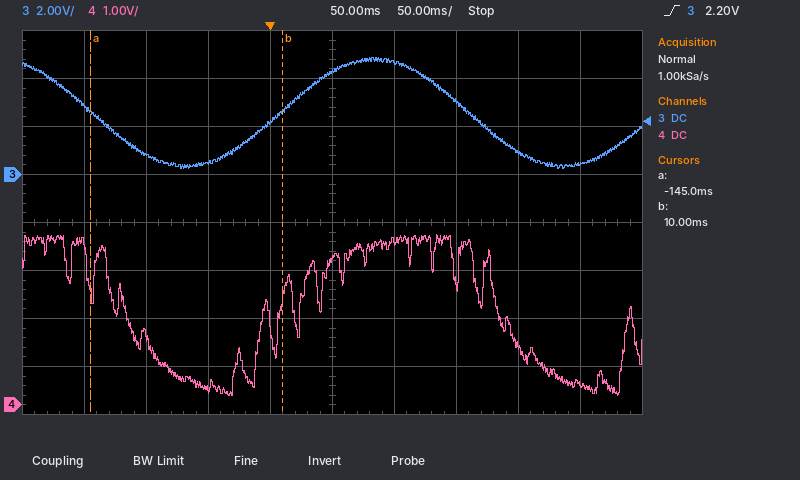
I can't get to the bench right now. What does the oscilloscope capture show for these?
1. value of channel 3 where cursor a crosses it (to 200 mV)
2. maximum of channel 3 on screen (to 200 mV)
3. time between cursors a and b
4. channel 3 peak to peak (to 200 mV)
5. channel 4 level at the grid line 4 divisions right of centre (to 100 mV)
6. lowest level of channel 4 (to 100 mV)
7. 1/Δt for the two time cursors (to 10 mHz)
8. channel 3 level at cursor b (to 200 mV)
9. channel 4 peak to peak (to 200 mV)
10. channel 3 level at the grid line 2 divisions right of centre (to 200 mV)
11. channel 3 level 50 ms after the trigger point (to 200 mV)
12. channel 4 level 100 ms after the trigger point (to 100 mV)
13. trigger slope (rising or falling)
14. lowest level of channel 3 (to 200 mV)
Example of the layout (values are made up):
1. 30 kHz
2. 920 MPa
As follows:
1. 2.6 V
2. 4.8 V
3. 155 ms
4. 4.6 V
5. 400 mV
6. 200 mV
7. 6.45 Hz
8. 2.6 V
9. 3.4 V
10. 3.0 V
11. 4.2 V
12. 3.4 V
13. rising
14. 200 mV
